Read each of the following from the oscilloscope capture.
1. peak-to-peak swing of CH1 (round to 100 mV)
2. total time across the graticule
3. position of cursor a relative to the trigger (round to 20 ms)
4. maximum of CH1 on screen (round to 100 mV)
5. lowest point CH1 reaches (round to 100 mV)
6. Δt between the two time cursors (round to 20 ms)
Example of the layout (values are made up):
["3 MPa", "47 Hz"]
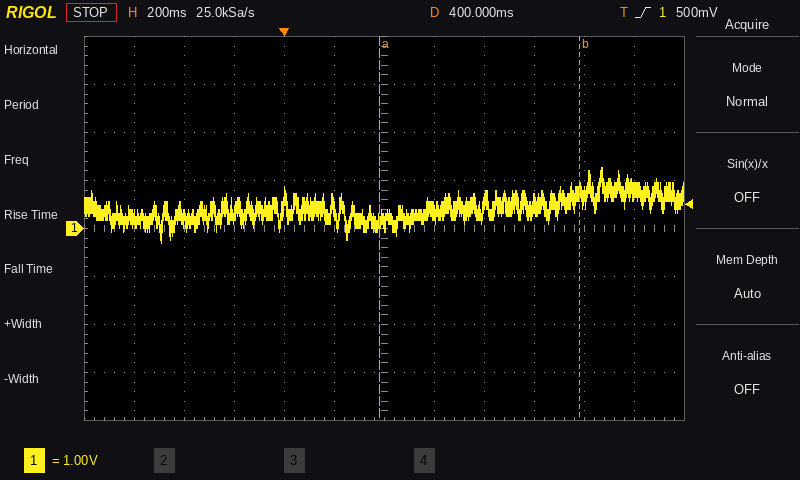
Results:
["1.6 V", "2.4 s", "+380 ms", "1.3 V", "-300 mV", "800 ms"]
